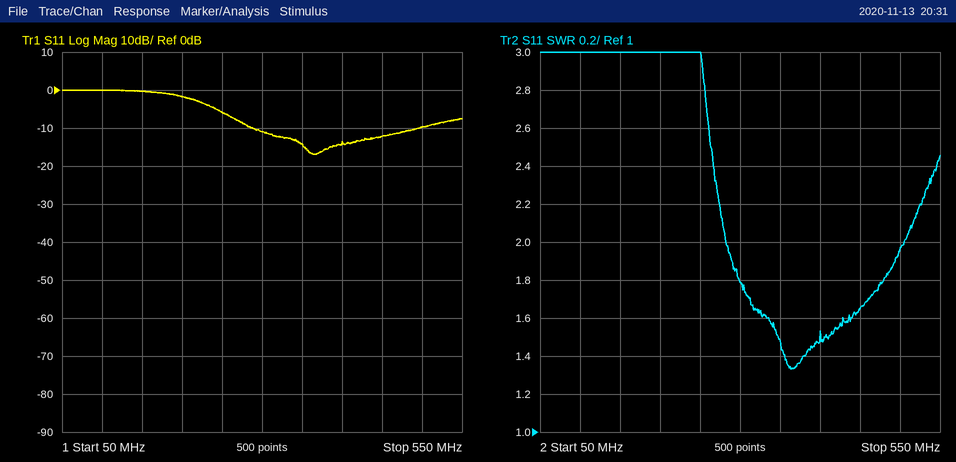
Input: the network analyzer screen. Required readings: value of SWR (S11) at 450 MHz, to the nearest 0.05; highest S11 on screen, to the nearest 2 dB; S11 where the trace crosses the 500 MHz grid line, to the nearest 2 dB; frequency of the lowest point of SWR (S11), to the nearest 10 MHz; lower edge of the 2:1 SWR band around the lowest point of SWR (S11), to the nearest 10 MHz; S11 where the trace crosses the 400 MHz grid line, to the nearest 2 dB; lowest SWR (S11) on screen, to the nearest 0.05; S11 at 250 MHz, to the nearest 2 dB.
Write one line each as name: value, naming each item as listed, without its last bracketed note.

value of SWR (S11) at 450 MHz, to the nearest 0.05: 1.65
highest S11 on screen, to the nearest 2 dB: 0 dB
S11 where the trace crosses the 500 MHz grid line, to the nearest 2 dB: -10 dB
frequency of the lowest point of SWR (S11), to the nearest 10 MHz: 360 MHz
lower edge of the 2:1 SWR band around the lowest point of SWR (S11), to the nearest 10 MHz: 280 MHz
S11 where the trace crosses the 400 MHz grid line, to the nearest 2 dB: -14 dB
lowest SWR (S11) on screen, to the nearest 0.05: 1.35
S11 at 250 MHz, to the nearest 2 dB: -6 dB
